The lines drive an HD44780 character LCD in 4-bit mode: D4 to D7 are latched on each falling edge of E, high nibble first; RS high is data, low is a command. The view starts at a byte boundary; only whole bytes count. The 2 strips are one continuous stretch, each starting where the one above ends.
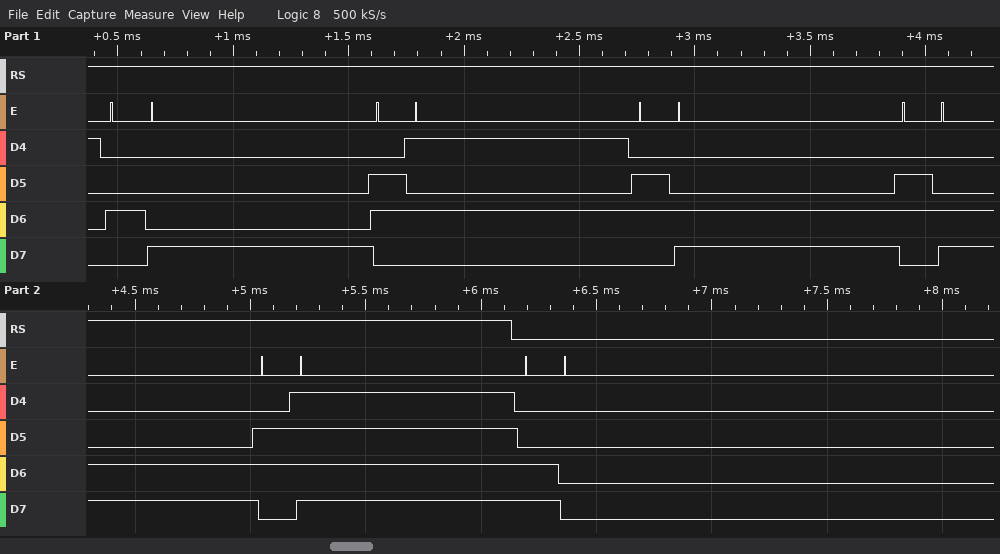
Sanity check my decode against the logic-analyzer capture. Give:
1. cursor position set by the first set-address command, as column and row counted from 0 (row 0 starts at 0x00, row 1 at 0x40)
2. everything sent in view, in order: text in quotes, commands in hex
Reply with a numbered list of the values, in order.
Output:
1. column 0, row 1
2. "Hello" 0xC0
